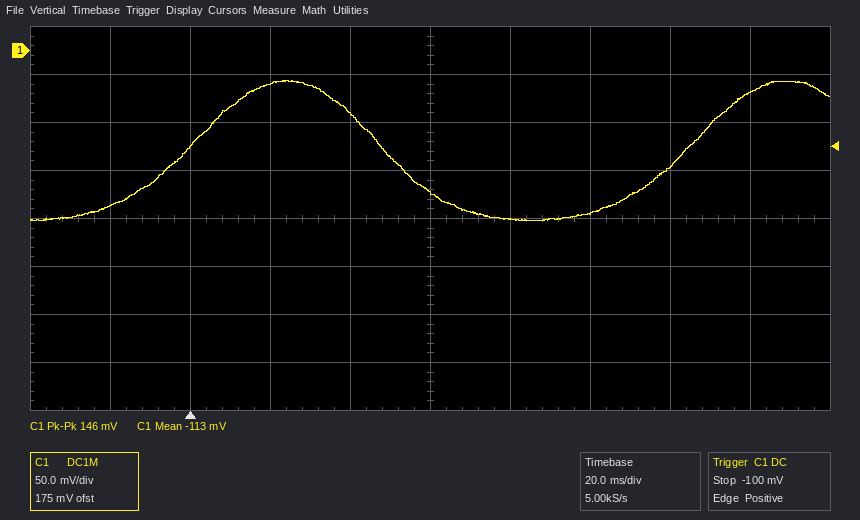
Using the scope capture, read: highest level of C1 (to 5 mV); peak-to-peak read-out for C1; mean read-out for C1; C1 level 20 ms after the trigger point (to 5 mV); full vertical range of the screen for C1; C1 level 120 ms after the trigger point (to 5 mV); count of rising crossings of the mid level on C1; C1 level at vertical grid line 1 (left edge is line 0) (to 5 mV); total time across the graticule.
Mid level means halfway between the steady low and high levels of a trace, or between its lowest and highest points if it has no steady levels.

-30 mV
146 mV
-113 mV
-35 mV
400 mV
-120 mV
2
-160 mV
200 ms
